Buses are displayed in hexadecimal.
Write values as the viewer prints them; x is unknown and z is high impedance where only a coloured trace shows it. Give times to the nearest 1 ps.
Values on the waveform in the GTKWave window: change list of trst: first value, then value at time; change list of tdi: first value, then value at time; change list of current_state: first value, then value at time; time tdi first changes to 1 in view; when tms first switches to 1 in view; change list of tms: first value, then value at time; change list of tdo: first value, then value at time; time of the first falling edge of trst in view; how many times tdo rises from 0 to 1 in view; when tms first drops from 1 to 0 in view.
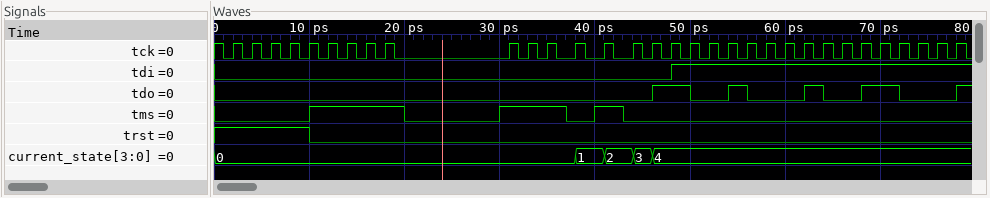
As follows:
1, 0 at 10 ps
0, 1 at 48 ps
0, 1 at 38 ps, 2 at 41 ps, 3 at 44 ps, 4 at 46 ps
48 ps
10 ps
0, 1 at 10 ps, 0 at 20 ps, 1 at 30 ps, 0 at 37 ps, 1 at 40 ps, 0 at 43 ps
0, 1 at 46 ps, 0 at 50 ps, 1 at 54 ps, 0 at 56 ps, 1 at 62 ps, 0 at 64 ps, 1 at 68 ps, 0 at 72 ps, 1 at 78 ps
10 ps
5
20 ps
